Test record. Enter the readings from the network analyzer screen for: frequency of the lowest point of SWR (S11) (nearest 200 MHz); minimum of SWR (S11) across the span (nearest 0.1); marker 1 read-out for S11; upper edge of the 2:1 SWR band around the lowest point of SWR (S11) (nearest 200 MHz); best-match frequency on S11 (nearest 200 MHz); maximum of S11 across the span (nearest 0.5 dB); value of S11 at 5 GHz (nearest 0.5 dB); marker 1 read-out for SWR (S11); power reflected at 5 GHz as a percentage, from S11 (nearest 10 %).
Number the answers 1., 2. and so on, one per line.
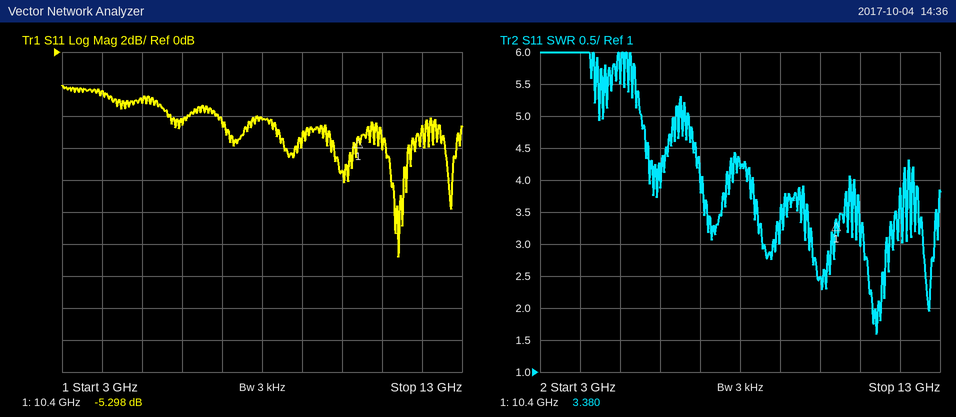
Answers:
1. 11.4 GHz
2. 1.6
3. -5.298 dB
4. 11.4 GHz
5. 11.4 GHz
6. -2.0 dB
7. -3.0 dB
8. 3.380
9. 50 %
